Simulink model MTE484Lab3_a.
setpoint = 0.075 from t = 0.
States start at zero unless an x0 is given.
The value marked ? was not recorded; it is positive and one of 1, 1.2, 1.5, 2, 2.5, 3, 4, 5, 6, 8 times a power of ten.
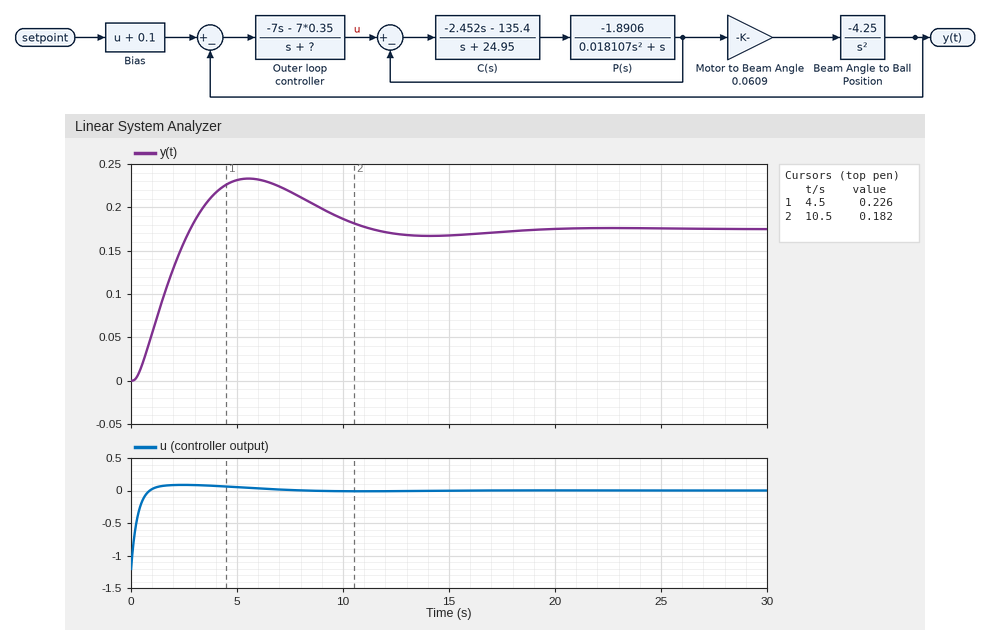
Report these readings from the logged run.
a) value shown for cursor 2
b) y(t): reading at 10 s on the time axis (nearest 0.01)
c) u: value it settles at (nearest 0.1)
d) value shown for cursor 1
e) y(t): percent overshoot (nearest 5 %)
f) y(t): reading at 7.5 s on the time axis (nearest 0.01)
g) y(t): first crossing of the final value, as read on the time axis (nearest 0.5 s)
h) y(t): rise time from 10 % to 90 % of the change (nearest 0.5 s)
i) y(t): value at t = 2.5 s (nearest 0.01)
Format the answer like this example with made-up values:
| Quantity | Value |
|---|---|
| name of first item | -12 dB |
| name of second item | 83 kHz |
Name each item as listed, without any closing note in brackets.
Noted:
| Quantity | Value |
|---|---|
| value shown for cursor 2 | 0.182 |
| y(t): reading at 10 s on the time axis | 0.19 |
| u: value it settles at | 0.0 |
| value shown for cursor 1 | 0.226 |
| y(t): percent overshoot | 35 % |
| y(t): reading at 7.5 s on the time axis | 0.22 |
| y(t): first crossing of the final value, as read on the time axis | 3.0 s |
| y(t): rise time from 10 % to 90 % of the change | 2.0 s |
| y(t): value at t = 2.5 s | 0.16 |
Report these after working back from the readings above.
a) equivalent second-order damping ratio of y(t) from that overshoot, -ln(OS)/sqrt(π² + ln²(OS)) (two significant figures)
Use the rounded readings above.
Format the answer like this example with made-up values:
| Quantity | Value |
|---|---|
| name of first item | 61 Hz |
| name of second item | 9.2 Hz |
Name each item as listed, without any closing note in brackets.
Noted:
| Quantity | Value |
|---|---|
| equivalent second-order damping ratio of y(t) from that overshoot, -ln(OS)/sqrt(π² + ln²(OS)) | 0.32 |
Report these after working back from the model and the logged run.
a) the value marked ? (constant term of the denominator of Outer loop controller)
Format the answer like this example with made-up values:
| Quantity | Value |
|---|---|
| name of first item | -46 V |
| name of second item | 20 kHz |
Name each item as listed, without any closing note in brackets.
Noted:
| Quantity | Value |
|---|---|
| the value marked ? | 4 |
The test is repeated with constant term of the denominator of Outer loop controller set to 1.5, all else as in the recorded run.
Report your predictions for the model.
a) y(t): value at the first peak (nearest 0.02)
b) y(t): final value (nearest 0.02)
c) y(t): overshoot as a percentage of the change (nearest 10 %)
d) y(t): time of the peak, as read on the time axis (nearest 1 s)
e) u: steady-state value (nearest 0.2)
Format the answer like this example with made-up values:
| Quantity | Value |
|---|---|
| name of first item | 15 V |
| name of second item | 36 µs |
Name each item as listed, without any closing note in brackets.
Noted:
| Quantity | Value |
|---|---|
| y(t): value at the first peak | 0.26 |
| y(t): final value | 0.18 |
| y(t): overshoot as a percentage of the change | 50 % |
| y(t): time of the peak, as read on the time axis | 3 s |
| u: steady-state value | 0.0 |
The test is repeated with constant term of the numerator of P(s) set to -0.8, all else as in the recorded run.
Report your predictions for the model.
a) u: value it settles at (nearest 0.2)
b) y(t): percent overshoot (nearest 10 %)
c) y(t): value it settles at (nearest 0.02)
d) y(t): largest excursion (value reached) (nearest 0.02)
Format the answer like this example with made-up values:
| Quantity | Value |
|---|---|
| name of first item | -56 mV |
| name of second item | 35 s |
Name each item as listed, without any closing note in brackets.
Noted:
| Quantity | Value |
|---|---|
| u: value it settles at | 0.0 |
| y(t): percent overshoot | 40 % |
| y(t): value it settles at | 0.18 |
| y(t): largest excursion (value reached) | 0.24 |
